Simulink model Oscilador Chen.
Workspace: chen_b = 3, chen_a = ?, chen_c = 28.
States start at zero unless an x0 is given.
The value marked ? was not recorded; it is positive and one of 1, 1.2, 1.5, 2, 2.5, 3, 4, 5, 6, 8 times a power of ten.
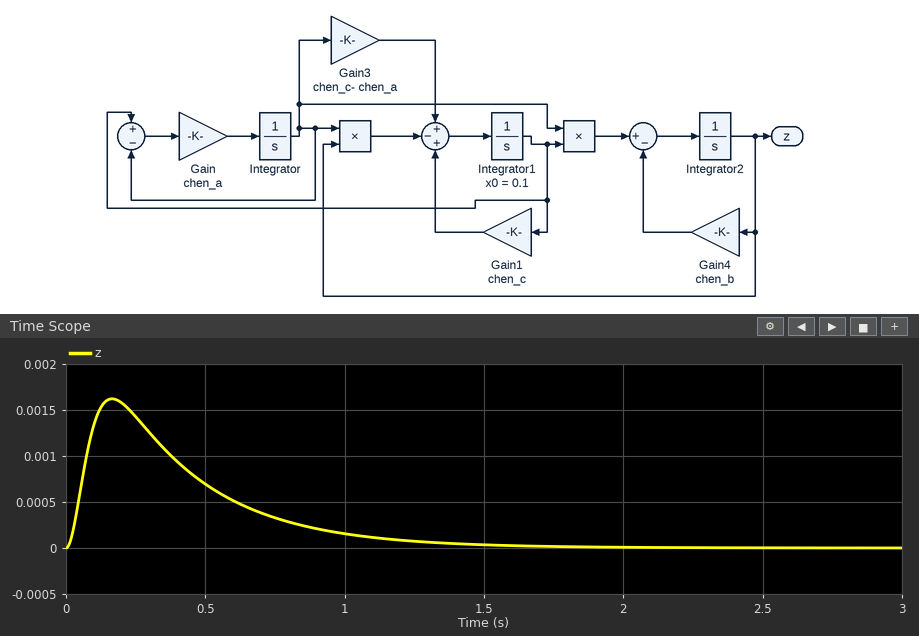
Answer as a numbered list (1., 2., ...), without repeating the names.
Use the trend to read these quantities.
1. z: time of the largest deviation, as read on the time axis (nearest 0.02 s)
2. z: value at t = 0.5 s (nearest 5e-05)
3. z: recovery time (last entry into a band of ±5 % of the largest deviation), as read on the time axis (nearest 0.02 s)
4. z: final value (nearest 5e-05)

1. 0.16 s
2. 0.00070
3. 1.22 s
4. 0.00000
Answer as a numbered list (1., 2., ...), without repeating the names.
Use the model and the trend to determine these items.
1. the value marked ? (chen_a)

1. 60
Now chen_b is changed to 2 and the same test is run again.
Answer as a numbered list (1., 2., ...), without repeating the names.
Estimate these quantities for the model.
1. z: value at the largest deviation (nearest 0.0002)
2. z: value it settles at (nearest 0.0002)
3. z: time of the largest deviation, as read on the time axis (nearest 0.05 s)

1. 0.0018
2. 0.0000
3. 0.20 s
